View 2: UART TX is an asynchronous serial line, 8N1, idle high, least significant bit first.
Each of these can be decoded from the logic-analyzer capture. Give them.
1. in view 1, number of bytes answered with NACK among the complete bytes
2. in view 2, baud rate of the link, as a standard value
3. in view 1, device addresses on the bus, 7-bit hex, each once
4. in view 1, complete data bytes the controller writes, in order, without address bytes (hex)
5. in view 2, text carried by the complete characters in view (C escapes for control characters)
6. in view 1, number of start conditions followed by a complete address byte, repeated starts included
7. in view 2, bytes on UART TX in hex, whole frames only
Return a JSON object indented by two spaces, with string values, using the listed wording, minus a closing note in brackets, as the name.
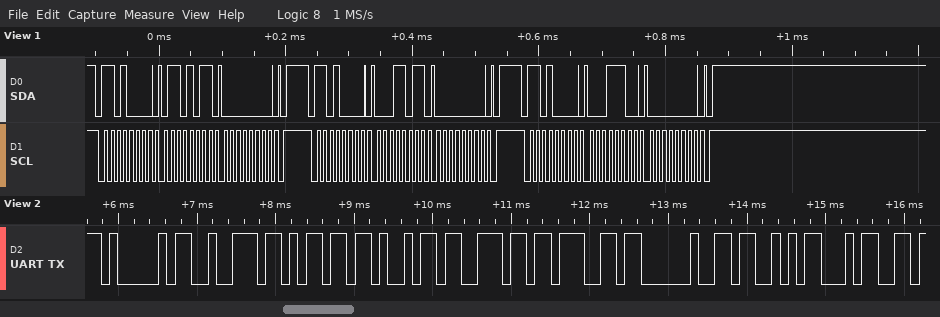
{
  "in view 1, number of bytes answered with NACK among the complete bytes": "0",
  "in view 2, baud rate of the link, as a standard value": "9600 baud",
  "in view 1, device addresses on the bus, 7-bit hex, each once": "0x68",
  "in view 1, complete data bytes the controller writes, in order, without address bytes": "6B 00 1B 00 1C 00",
  "in view 2, text carried by the complete characters in view": "\"Arming S4\"",
  "in view 1, number of start conditions followed by a complete address byte, repeated starts included": "3",
  "in view 2, bytes on UART TX in hex, whole frames only": "41 72 6D 69 6E 67 20 53 34"
}
